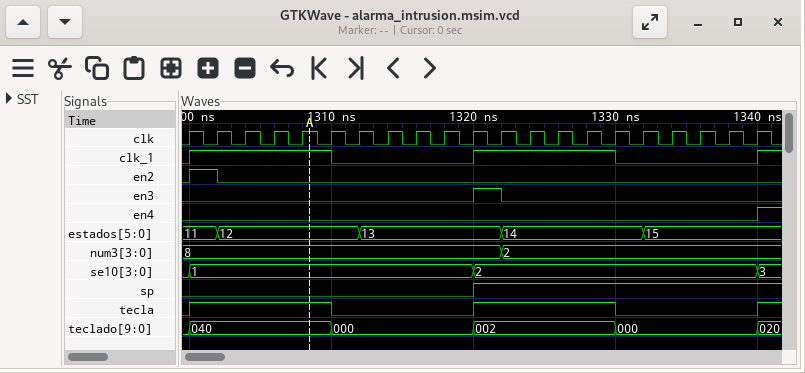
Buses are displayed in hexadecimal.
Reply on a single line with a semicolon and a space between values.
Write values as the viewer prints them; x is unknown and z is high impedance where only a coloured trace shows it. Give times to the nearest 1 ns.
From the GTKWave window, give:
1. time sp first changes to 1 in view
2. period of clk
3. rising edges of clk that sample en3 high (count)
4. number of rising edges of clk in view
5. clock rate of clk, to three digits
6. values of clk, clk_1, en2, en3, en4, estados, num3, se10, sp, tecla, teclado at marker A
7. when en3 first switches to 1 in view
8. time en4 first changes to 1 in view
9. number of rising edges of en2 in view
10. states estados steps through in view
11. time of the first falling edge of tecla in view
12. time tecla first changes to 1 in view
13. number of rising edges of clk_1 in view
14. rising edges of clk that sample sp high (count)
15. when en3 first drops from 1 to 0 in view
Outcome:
1320 ns; 2 ns; 1; 21; 500 MHz; clk=1, clk_1=1, en2=0, en3=0, en4=0, estados=12, num3=8, se10=1, sp=0, tecla=1, teclado=040; 1320 ns; 1340 ns; 1; 11, 12, 13, 14, 15; 1310 ns; 1300 ns; 3; 10; 1322 ns
